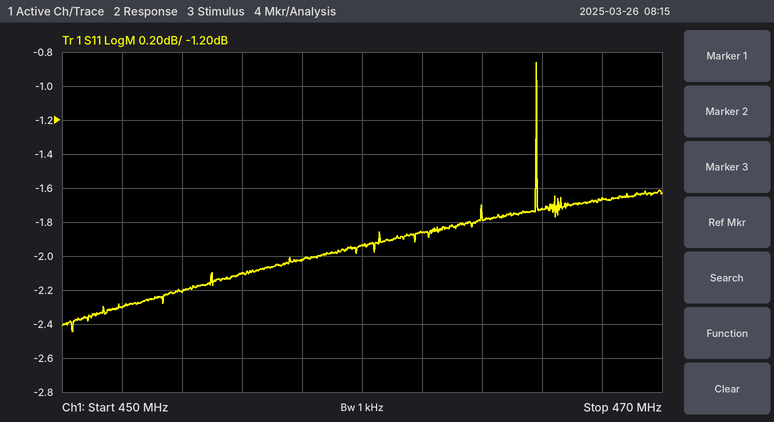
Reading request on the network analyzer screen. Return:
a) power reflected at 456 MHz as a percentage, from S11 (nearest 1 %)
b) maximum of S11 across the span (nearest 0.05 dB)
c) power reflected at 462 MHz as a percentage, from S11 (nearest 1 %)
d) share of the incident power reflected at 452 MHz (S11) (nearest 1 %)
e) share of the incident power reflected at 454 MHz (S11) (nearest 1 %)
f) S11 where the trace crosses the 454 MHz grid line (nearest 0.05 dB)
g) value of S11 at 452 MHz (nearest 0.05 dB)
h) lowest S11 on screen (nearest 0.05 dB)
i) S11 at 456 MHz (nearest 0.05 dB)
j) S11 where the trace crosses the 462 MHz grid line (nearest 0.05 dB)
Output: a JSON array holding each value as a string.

["62 %", "-0.85 dB", "65 %", "59 %", "60 %", "-2.20 dB", "-2.30 dB", "-2.45 dB", "-2.10 dB", "-1.85 dB"]
